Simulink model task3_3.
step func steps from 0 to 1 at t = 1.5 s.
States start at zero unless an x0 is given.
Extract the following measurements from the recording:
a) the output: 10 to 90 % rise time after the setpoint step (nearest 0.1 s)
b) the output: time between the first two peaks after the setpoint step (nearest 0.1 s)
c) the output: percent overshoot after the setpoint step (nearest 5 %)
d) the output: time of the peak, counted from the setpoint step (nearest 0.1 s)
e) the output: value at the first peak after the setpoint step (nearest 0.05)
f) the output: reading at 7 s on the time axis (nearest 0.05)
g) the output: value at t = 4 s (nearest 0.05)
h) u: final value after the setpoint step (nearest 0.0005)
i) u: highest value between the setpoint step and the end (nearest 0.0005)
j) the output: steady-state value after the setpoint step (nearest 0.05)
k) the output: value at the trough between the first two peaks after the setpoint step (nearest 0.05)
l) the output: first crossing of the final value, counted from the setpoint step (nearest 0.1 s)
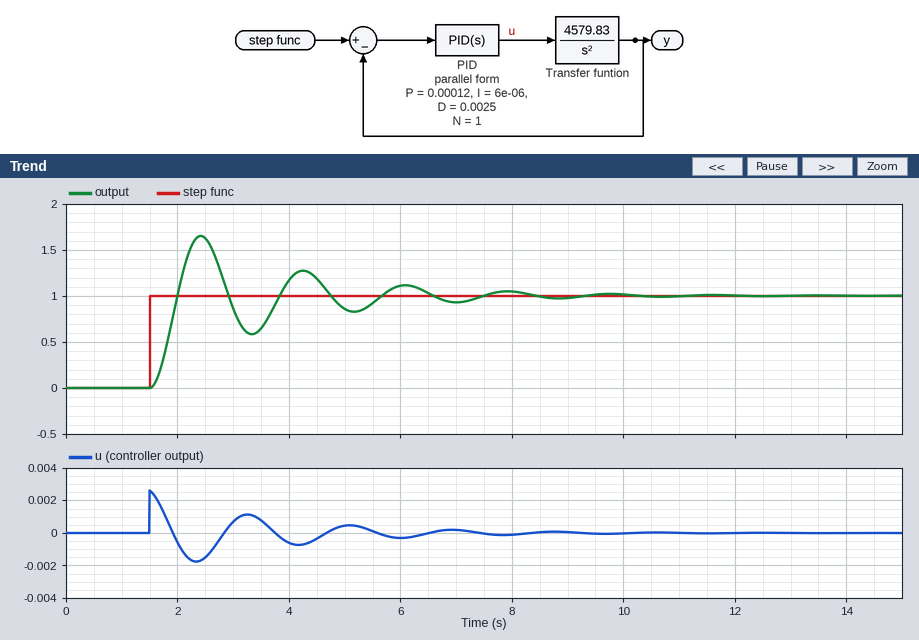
0.3 s
1.8 s
65 %
0.9 s
1.65
0.95
1.15
0.0000
0.0025
1.00
0.60
0.5 s
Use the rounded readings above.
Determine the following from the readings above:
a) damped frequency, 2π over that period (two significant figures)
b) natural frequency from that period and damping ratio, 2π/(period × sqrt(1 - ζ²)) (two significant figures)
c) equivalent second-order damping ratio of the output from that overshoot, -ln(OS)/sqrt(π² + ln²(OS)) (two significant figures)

3.5 rad/s
3.5 rad/s
0.14
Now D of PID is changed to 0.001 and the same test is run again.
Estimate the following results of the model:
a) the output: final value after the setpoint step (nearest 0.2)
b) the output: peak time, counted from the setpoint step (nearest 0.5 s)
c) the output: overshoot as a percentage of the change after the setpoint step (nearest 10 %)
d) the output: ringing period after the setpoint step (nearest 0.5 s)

1.0
1.5 s
60 %
3.0 s
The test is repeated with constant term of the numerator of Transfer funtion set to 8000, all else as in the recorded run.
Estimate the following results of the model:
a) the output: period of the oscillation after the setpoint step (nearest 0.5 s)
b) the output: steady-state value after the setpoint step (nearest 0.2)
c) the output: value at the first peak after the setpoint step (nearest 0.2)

1.5 s
1.0
1.8
